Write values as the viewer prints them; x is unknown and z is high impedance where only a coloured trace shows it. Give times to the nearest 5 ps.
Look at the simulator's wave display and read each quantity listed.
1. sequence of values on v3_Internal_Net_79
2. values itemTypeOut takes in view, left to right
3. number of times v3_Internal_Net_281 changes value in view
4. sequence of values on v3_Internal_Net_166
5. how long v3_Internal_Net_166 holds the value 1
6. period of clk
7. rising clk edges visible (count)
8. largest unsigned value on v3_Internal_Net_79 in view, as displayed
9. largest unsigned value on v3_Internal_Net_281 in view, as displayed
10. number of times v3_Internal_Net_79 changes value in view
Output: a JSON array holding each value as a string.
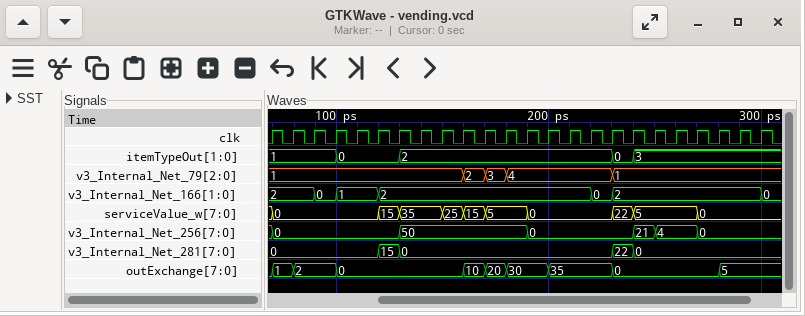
["1, 2, 3, 4, 1", "1, 0, 2, 0, 3", "4", "2, 0, 1, 2, 0, 2, 0", "20 ps", "10 ps", "24", "4", "22", "4"]
